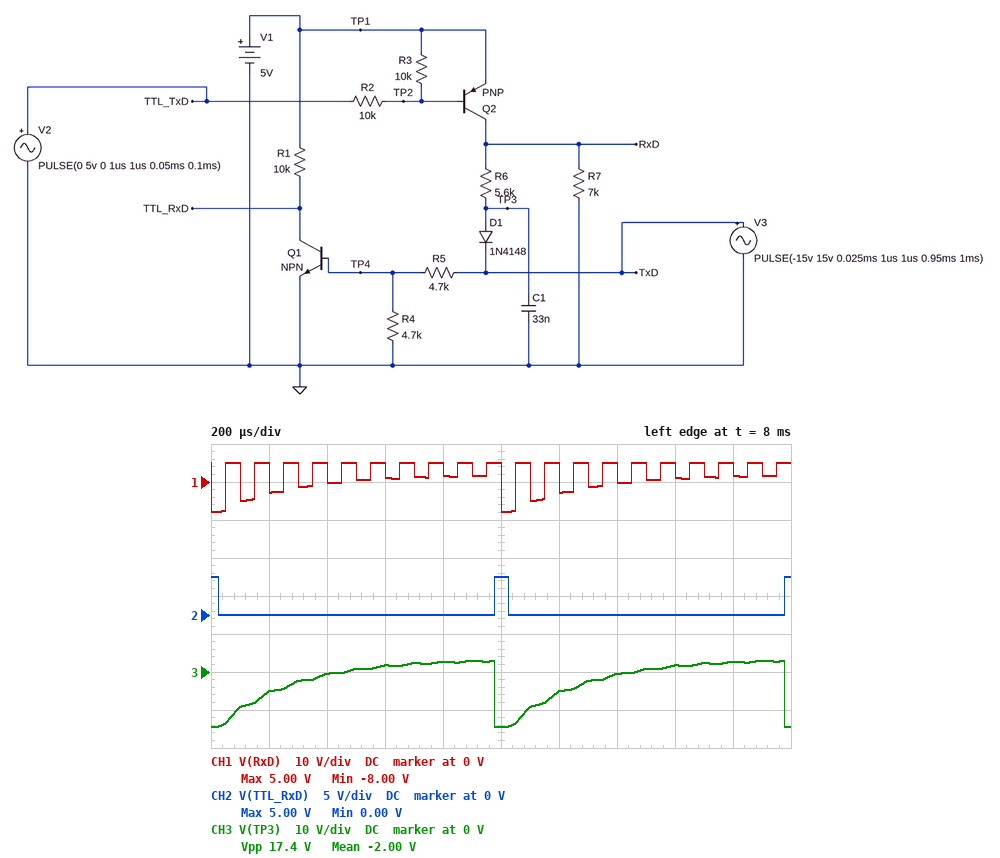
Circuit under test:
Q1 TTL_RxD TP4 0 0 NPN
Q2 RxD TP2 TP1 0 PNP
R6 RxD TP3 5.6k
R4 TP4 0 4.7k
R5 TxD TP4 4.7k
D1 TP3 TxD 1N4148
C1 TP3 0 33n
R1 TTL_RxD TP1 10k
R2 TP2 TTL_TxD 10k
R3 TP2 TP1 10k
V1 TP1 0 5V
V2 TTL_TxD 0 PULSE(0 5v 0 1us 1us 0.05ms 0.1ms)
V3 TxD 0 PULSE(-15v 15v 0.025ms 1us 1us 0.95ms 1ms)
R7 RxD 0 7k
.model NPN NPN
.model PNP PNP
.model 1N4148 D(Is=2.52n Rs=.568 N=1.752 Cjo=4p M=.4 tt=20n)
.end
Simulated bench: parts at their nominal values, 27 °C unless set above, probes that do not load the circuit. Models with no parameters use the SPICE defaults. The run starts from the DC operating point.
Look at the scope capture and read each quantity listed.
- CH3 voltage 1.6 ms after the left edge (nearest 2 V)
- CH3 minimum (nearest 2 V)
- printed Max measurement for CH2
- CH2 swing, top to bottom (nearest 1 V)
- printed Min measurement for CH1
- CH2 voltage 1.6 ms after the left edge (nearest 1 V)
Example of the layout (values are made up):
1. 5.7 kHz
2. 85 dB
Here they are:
1. 2 V
2. -14 V
3. 5.00 V
4. 5 V
5. -8.00 V
6. 0 V
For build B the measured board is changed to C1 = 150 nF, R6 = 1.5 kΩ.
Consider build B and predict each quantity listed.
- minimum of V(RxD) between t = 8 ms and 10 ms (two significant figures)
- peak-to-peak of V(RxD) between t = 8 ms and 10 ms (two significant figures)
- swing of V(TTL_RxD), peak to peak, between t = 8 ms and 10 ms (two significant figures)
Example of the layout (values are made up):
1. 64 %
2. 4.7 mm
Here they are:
1. -12 V
2. 17 V
3. 5.0 V
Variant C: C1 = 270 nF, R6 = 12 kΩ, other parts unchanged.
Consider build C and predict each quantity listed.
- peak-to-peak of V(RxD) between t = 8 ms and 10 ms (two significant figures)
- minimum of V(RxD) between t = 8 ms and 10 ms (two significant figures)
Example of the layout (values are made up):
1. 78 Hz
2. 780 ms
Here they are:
1. 10 V
2. -5.3 V
